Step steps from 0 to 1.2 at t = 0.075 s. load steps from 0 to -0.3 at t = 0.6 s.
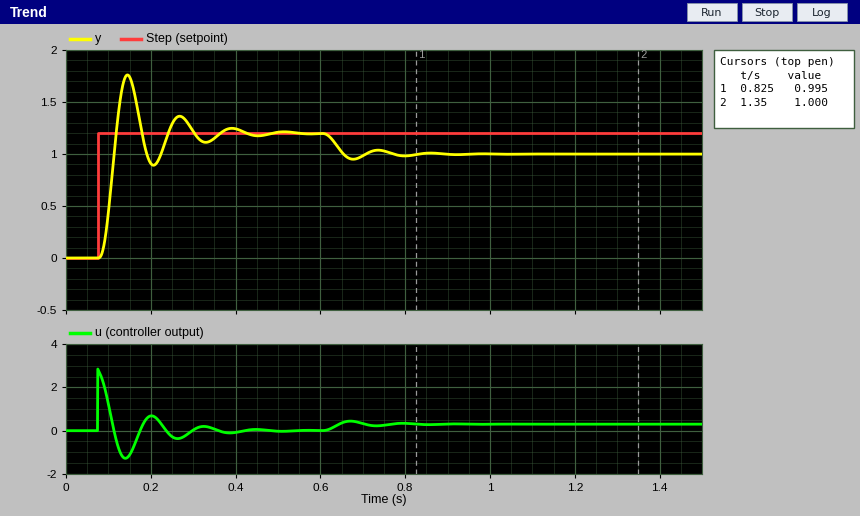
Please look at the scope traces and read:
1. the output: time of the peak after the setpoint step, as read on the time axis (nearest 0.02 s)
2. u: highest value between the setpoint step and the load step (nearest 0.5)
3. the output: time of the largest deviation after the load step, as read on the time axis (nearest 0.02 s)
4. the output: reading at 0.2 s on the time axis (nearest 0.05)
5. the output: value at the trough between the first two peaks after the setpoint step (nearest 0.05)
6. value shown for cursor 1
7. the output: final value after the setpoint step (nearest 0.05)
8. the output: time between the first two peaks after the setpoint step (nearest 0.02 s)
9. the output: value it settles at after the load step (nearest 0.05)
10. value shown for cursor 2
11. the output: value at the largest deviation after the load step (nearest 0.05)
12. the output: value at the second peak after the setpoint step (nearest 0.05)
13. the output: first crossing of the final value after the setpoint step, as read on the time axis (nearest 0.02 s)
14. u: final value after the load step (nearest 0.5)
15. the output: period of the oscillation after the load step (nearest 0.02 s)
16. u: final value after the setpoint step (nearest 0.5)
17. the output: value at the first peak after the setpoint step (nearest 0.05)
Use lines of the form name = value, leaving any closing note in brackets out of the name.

the output: time of the peak after the setpoint step, as read on the time axis = 0.14 s
u: highest value between the setpoint step and the load step = 3.0
the output: time of the largest deviation after the load step, as read on the time axis = 0.68 s
the output: reading at 0.2 s on the time axis = 0.90
the output: value at the trough between the first two peaks after the setpoint step = 0.90
value shown for cursor 1 = 0.995
the output: final value after the setpoint step = 1.20
the output: time between the first two peaks after the setpoint step = 0.12 s
the output: value it settles at after the load step = 1.00
value shown for cursor 2 = 1.000
the output: value at the largest deviation after the load step = 0.95
the output: value at the second peak after the setpoint step = 1.35
the output: first crossing of the final value after the setpoint step, as read on the time axis = 0.12 s
u: final value after the load step = 0.5
the output: period of the oscillation after the load step = 0.12 s
u: final value after the setpoint step = 0.0
the output: value at the first peak after the setpoint step = 1.75
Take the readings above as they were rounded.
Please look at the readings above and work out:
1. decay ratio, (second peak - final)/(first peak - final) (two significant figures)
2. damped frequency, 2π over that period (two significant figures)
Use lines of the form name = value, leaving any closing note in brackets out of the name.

decay ratio, (second peak - final)/(first peak - final) = 0.27
damped frequency, 2π over that period = 52 rad/s
